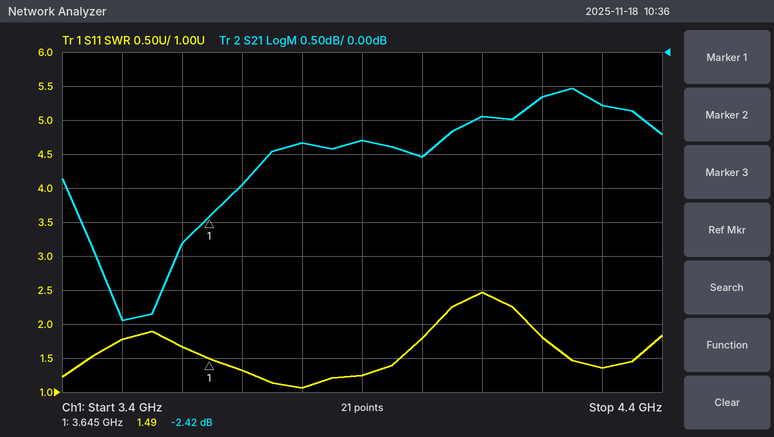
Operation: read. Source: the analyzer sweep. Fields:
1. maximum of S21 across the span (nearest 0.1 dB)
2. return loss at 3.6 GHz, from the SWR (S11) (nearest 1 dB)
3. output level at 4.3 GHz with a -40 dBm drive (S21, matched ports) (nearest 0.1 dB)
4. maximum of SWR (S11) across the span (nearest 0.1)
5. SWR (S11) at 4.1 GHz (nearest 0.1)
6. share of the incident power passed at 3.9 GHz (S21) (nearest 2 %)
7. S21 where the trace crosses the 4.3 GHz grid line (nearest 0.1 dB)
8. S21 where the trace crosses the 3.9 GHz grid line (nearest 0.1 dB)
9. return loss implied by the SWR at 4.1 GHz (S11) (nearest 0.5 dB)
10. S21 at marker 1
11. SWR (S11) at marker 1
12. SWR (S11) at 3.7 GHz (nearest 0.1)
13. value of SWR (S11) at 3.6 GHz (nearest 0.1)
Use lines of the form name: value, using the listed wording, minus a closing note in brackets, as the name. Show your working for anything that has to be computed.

maximum of S21 across the span: -0.5 dB
return loss at 3.6 GHz, from the SWR (S11): −20 log10((1.7 − 1)/(1.7 + 1)) ≈ 12 dB
output level at 4.3 GHz with a -40 dBm drive (S21, matched ports): -40 dBm + (-0.8 dB) = -40.8 dBm
maximum of SWR (S11) across the span: 2.5
SWR (S11) at 4.1 GHz: 2.5
share of the incident power passed at 3.9 GHz (S21): 10^(-1.3/10) ≈ 74 %
S21 where the trace crosses the 4.3 GHz grid line: -0.8 dB
S21 where the trace crosses the 3.9 GHz grid line: -1.3 dB
return loss implied by the SWR at 4.1 GHz (S11): −20 log10((2.5 − 1)/(2.5 + 1)) ≈ 7.36 dB, so 7.5 dB to the nearest 0.5 dB
S21 at marker 1: -2.42 dB
SWR (S11) at marker 1: 1.49
SWR (S11) at 3.7 GHz: 1.3
value of SWR (S11) at 3.6 GHz: 1.7
